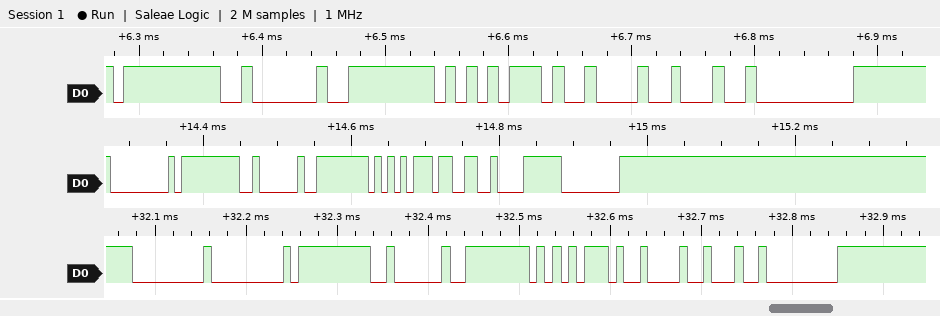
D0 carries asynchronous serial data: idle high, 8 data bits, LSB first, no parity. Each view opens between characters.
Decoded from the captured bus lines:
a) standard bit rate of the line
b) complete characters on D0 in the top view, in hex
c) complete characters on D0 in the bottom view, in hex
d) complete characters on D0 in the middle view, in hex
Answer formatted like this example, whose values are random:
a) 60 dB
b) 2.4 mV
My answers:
a) 115200 baud
b) FF, 02, FE, D5, 09, 22, 00
c) 00, 00, FF, 02, FE, D5, 09, 22, 00
d) 00, FF, 02, FE, D5, 33, F8, 00
